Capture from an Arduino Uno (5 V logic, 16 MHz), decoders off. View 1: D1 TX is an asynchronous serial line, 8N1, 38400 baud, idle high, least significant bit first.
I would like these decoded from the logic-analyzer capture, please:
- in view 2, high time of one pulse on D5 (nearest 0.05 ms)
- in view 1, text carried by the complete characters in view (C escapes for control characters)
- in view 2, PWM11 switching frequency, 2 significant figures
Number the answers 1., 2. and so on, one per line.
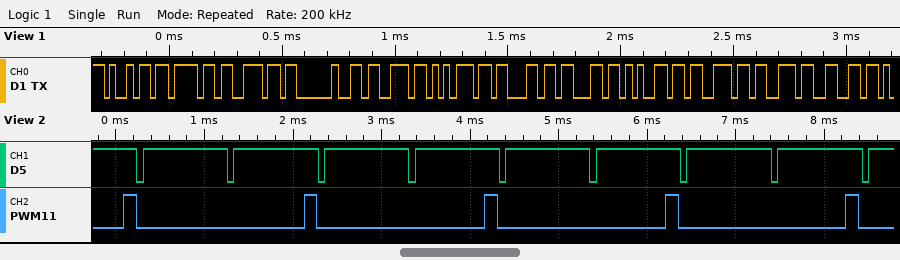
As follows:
1. 0.95 ms
2. "ion successf"
3. 490 Hz
